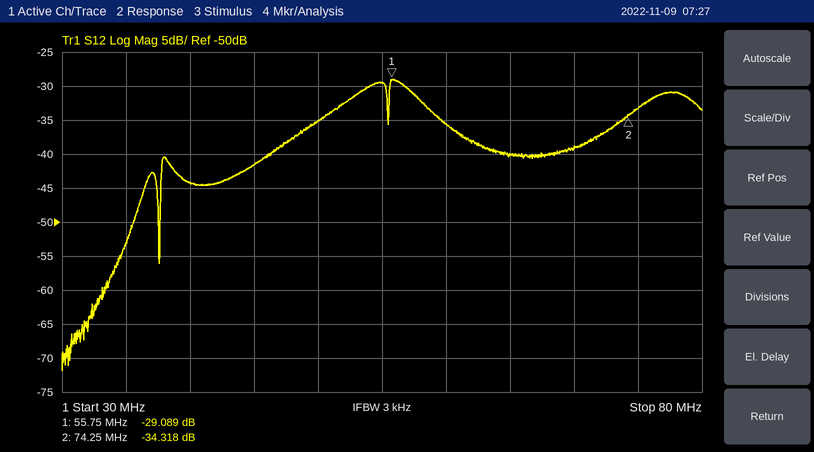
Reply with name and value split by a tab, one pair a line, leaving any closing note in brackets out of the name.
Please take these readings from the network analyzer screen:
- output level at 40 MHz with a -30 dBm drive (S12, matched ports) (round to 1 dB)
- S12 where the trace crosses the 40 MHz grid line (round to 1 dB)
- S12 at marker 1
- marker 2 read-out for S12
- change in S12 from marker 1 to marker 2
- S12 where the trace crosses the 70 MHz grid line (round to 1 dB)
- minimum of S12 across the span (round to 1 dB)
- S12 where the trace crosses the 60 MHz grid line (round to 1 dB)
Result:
output level at 40 MHz with a -30 dBm drive (S12, matched ports)	-74 dBm
S12 where the trace crosses the 40 MHz grid line	-44 dB
S12 at marker 1	-29.089 dB
marker 2 read-out for S12	-34.318 dB
change in S12 from marker 1 to marker 2	-5.229 dB
S12 where the trace crosses the 70 MHz grid line	-39 dB
minimum of S12 across the span	-72 dB
S12 where the trace crosses the 60 MHz grid line	-36 dB
